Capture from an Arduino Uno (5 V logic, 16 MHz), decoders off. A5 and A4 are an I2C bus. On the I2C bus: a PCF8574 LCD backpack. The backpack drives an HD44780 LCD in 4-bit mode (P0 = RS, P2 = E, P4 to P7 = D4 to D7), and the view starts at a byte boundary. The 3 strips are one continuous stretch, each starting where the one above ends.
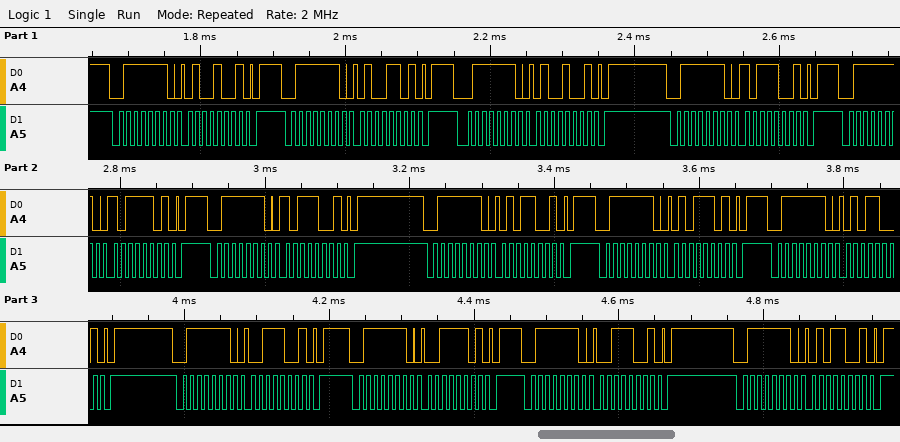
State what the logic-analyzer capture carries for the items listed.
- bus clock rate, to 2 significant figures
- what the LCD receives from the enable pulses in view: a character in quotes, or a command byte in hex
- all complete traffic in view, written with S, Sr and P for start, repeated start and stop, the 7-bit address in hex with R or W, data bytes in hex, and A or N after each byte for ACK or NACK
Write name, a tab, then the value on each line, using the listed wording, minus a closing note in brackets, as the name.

bus clock rate, to 2 significant figures	100 kHz
what the LCD receives from the enable pulses in view: a character in quotes, or a command byte in hex	'K' 'S'
all complete traffic in view, written with S, Sr and P for start, repeated start and stop, the 7-bit address in hex with R or W, data bytes in hex, and A or N after each byte for ACK or NACK	S 3FW A 49 A P S 3FW A 4D A P S 3FW A 49 A P S 3FW A B9 A P S 3FW A BD A P S 3FW A B9 A P S 3FW A 59 A P S 3FW A 5D A P S 3FW A 59 A P S 3FW A 39 A P S 3FW A 3D A P S 3FW A 39 A P S 3FW A 59 A P
